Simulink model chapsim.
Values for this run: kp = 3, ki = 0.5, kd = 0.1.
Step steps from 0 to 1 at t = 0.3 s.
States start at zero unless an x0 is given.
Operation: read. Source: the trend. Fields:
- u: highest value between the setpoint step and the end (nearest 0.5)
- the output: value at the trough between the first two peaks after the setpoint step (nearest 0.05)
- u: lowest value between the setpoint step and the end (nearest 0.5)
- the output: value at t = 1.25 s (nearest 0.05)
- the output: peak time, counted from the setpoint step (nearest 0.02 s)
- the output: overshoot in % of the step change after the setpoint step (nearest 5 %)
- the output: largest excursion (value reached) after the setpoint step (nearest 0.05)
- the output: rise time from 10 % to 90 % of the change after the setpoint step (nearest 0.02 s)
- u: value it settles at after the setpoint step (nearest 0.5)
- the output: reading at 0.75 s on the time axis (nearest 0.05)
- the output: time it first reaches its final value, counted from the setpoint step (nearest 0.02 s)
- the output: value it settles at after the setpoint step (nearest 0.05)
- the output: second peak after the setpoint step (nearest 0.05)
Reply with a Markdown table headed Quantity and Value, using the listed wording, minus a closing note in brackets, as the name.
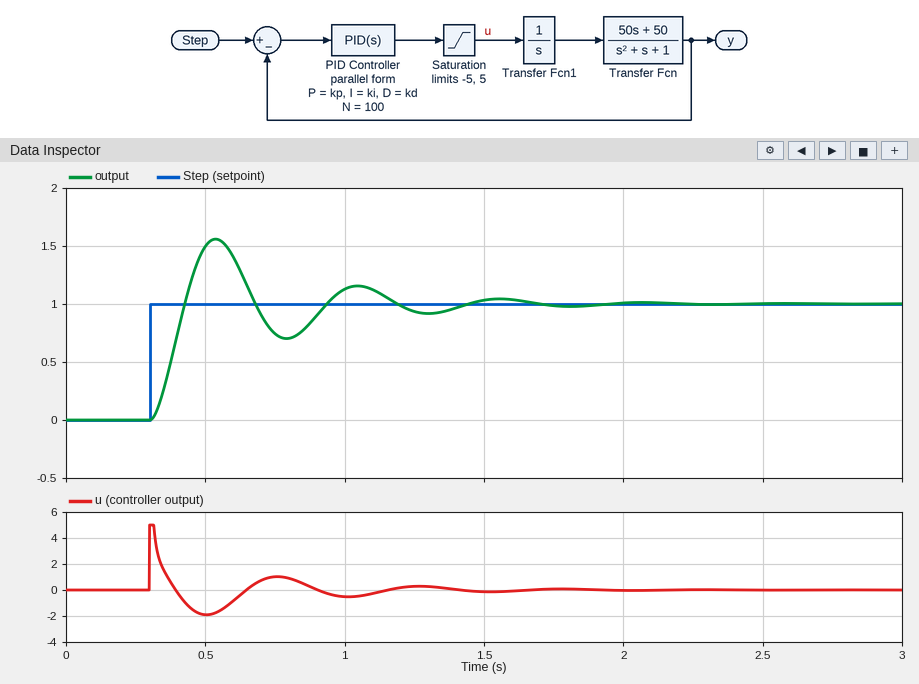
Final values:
| Quantity | Value |
|---|---|
| u: highest value between the setpoint step and the end | 5.0 |
| the output: value at the trough between the first two peaks after the setpoint step | 0.70 |
| u: lowest value between the setpoint step and the end | -2.0 |
| the output: value at t = 1.25 s | 0.95 |
| the output: peak time, counted from the setpoint step | 0.24 s |
| the output: overshoot in % of the step change after the setpoint step | 55 % |
| the output: largest excursion (value reached) after the setpoint step | 1.55 |
| the output: rise time from 10 % to 90 % of the change after the setpoint step | 0.08 s |
| u: value it settles at after the setpoint step | 0.0 |
| the output: reading at 0.75 s on the time axis | 0.75 |
| the output: time it first reaches its final value, counted from the setpoint step | 0.12 s |
| the output: value it settles at after the setpoint step | 1.00 |
| the output: second peak after the setpoint step | 1.15 |
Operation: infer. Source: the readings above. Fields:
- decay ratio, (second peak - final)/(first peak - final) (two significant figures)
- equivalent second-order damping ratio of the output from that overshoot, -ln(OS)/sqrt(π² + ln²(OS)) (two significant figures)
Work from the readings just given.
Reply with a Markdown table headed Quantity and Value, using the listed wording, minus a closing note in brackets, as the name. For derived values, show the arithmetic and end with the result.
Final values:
| Quantity | Value |
|---|---|
| decay ratio, (second peak - final)/(first peak - final) | (1.15 - 1) / (1.55 - 1) = 0.27 |
| equivalent second-order damping ratio of the output from that overshoot, -ln(OS)/sqrt(π² + ln²(OS)) | ln(0.55) = -0.598; 0.598 / sqrt(9.870 + 0.357) = 0.19 |
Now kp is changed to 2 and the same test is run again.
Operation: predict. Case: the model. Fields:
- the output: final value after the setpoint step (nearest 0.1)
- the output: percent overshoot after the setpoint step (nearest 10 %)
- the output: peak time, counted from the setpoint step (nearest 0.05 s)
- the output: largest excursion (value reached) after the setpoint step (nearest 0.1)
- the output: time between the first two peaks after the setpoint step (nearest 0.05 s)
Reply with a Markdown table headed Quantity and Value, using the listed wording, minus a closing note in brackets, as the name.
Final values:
| Quantity | Value |
|---|---|
| the output: final value after the setpoint step | 1.0 |
| the output: percent overshoot after the setpoint step | 50 % |
| the output: peak time, counted from the setpoint step | 0.30 s |
| the output: largest excursion (value reached) after the setpoint step | 1.5 |
| the output: time between the first two peaks after the setpoint step | 0.65 s |
